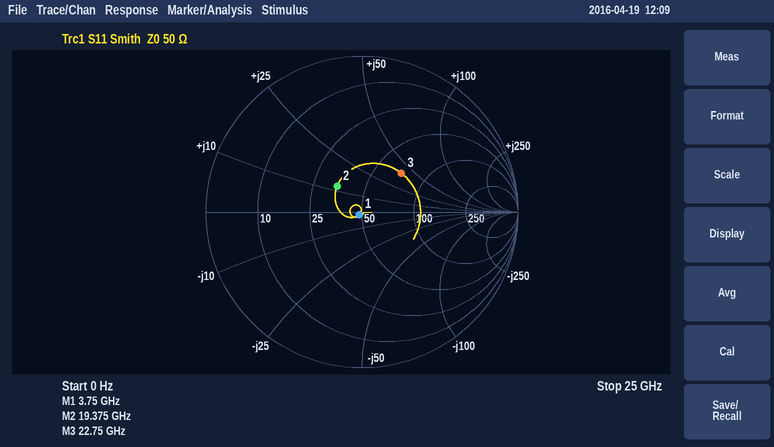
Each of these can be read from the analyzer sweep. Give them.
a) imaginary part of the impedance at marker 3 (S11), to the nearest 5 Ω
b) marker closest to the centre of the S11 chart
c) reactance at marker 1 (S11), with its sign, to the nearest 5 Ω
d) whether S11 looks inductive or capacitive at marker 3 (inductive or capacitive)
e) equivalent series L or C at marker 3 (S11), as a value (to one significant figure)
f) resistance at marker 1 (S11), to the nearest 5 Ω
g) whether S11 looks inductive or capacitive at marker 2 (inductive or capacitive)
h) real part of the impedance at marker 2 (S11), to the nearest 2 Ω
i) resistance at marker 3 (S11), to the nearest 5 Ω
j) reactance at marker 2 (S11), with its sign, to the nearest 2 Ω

+40 Ω
marker 1
0 Ω
inductive
300 pH
50 Ω
inductive
34 Ω
70 Ω
+12 Ω
